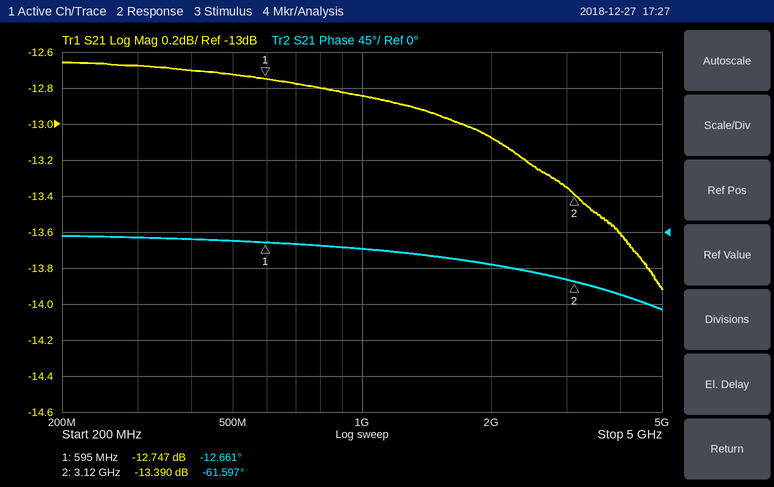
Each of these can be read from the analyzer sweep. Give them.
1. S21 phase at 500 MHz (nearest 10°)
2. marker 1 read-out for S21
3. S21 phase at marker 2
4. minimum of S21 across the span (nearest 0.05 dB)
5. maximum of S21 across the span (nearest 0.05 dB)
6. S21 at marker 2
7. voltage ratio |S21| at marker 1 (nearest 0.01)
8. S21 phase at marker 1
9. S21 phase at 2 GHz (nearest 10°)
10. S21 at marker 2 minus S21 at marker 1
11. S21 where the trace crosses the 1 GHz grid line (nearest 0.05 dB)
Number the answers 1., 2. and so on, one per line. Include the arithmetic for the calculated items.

1. -10°
2. -12.747 dB
3. -61.597°
4. -13.90 dB
5. -12.65 dB
6. -13.390 dB
7. 10^(-12.747/20) ≈ 0.23
8. -12.661°
9. -40°
10. -13.39 − (-12.747) = -0.643 dB
11. -12.85 dB
